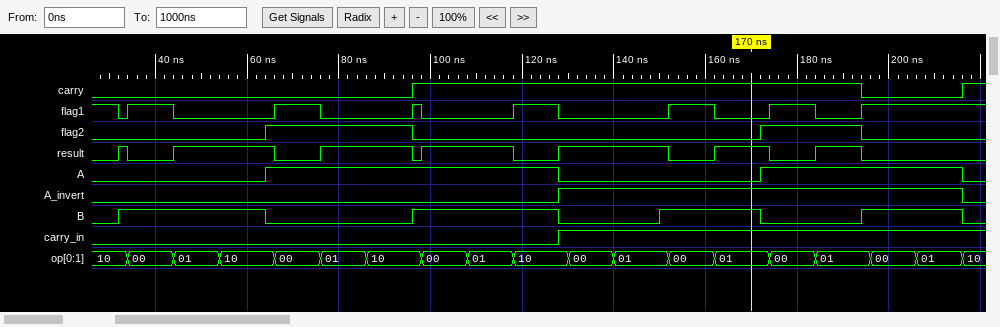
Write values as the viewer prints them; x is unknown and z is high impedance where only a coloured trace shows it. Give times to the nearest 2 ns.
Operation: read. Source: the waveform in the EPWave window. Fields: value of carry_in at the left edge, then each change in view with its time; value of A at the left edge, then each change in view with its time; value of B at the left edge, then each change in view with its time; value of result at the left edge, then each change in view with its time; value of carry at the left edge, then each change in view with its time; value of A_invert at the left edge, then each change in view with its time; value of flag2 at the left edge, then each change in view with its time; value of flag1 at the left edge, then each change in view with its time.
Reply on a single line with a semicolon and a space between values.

0, 1 at 128 ns; 0, 1 at 64 ns, 0 at 128 ns, 1 at 172 ns, 0 at 216 ns; 0, 1 at 32 ns, 0 at 64 ns, 1 at 96 ns, 0 at 128 ns, 1 at 150 ns, 0 at 172 ns, 1 at 194 ns, 0 at 216 ns; 0, 1 at 32 ns, 0 at 34 ns, 1 at 44 ns, 0 at 66 ns, 1 at 76 ns, 0 at 96 ns, 1 at 98 ns, 0 at 118 ns, 1 at 128 ns, 0 at 152 ns, 1 at 162 ns, 0 at 174 ns, 1 at 184 ns, 0 at 194 ns; 0, 1 at 96 ns, 0 at 194 ns, 1 at 216 ns; 0, 1 at 128 ns, 0 at 216 ns; 0, 1 at 64 ns, 0 at 96 ns, 1 at 172 ns, 0 at 194 ns; 1, 0 at 32 ns, 1 at 34 ns, 0 at 44 ns, 1 at 66 ns, 0 at 76 ns, 1 at 96 ns, 0 at 98 ns, 1 at 118 ns, 0 at 128 ns, 1 at 152 ns, 0 at 162 ns, 1 at 174 ns, 0 at 184 ns, 1 at 194 ns
